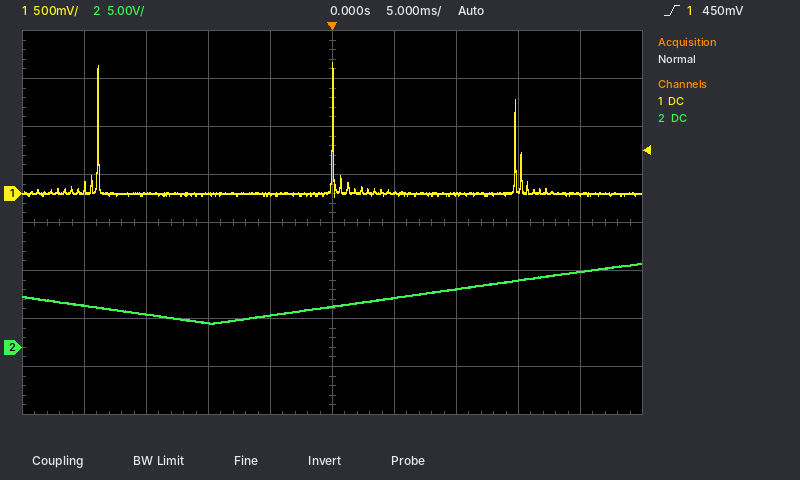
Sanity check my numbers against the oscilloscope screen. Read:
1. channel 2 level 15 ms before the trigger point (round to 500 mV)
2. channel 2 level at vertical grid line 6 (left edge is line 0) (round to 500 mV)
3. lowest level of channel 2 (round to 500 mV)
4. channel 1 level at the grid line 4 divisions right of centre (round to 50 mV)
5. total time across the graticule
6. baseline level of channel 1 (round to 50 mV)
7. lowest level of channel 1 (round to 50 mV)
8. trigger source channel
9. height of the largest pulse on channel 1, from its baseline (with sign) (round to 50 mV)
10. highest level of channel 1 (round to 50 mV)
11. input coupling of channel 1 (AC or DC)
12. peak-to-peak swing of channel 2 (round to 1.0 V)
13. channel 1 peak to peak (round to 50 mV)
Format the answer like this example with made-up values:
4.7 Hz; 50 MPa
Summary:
3.5 V; 5.0 V; 2.5 V; 0 mV; 50 ms; 0 mV; -50 mV; channel 1; +1.35 V; 1.35 V; DC; 6.0 V; 1.40 V
